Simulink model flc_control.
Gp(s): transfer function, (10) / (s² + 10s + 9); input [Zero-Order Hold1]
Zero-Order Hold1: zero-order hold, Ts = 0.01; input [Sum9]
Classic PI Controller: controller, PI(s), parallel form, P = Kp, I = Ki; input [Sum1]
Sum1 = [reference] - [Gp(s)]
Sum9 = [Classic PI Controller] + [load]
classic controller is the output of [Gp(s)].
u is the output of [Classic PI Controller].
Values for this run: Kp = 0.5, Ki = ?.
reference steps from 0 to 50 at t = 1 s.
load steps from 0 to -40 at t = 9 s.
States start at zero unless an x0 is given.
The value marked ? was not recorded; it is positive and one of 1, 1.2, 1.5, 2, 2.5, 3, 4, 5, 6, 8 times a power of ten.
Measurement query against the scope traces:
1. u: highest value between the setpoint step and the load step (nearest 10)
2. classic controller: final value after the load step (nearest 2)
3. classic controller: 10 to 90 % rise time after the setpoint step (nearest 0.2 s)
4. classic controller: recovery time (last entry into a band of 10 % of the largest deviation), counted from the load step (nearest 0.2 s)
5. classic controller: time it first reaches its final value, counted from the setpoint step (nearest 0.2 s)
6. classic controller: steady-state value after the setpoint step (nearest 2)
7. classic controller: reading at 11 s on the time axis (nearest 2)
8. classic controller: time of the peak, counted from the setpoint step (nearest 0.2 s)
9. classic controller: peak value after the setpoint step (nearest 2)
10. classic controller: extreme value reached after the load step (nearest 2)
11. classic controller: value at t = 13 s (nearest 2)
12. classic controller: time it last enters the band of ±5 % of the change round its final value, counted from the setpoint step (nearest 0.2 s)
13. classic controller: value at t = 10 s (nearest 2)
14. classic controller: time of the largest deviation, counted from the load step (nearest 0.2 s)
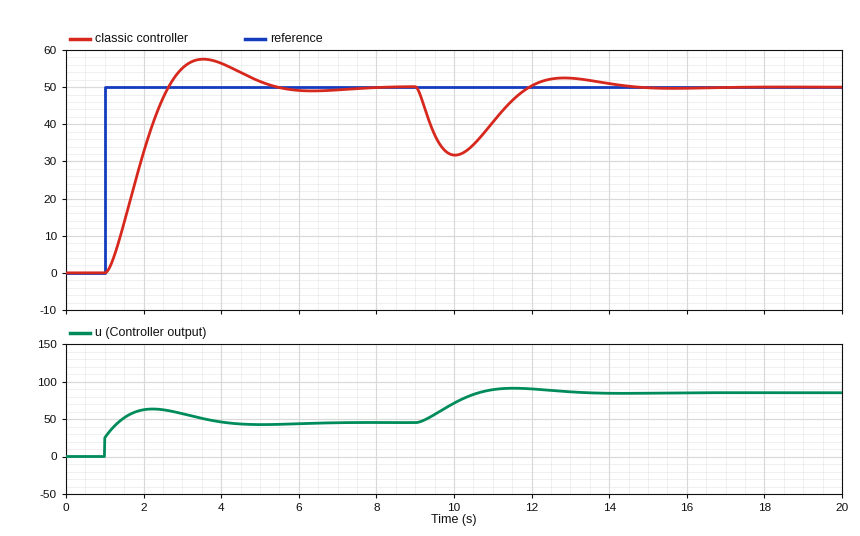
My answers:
60
50
1.2 s
4.4 s
1.6 s
50
40
2.6 s
58
32
52
3.8 s
32
1.0 s
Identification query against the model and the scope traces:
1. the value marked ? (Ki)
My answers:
1.5
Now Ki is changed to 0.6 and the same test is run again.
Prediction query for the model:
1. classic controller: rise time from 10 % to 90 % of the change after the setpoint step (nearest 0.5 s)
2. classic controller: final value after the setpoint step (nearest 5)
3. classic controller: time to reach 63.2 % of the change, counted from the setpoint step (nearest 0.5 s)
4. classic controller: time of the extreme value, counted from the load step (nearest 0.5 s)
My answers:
3.0 s
50
1.5 s
1.5 s
